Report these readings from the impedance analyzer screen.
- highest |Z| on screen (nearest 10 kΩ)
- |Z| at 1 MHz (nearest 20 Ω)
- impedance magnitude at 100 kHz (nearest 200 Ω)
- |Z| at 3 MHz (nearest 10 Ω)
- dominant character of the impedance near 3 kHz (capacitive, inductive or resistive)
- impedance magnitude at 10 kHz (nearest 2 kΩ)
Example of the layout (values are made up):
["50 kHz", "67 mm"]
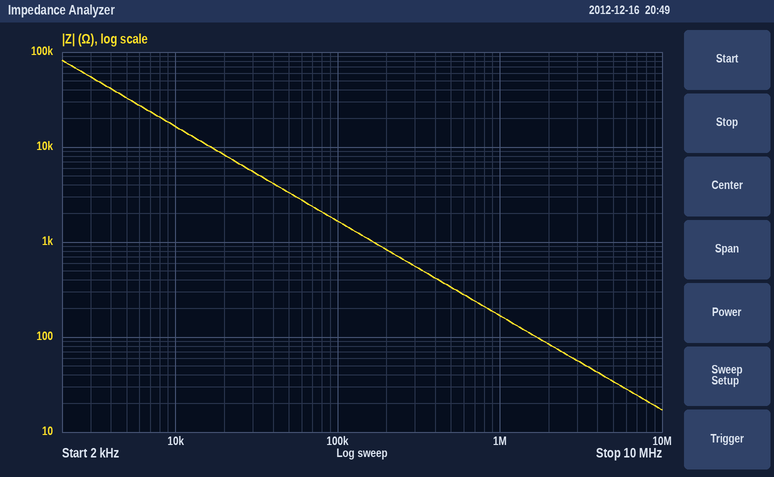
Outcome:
["80 kΩ", "160 Ω", "1.6 kΩ", "60 Ω", "capacitive", "16 kΩ"]
